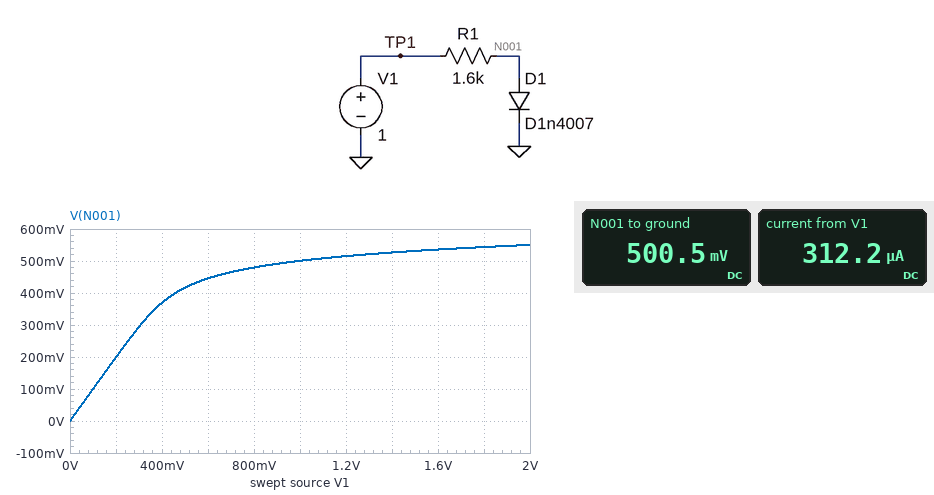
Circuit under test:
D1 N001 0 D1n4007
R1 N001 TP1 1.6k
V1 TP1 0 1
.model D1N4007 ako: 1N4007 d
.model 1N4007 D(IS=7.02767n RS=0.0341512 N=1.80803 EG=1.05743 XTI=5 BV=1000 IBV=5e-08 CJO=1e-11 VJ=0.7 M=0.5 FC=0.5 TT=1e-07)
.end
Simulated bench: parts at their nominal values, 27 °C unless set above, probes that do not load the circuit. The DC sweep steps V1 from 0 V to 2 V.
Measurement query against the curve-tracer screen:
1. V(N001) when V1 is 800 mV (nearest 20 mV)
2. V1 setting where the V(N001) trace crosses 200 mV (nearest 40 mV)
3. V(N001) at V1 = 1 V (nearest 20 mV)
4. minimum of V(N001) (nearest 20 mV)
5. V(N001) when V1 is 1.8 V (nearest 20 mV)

480 mV
200 mV
500 mV
0 V
540 mV
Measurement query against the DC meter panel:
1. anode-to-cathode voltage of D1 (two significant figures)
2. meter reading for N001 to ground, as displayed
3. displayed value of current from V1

500 mV
500.5 mV
312.2 µA
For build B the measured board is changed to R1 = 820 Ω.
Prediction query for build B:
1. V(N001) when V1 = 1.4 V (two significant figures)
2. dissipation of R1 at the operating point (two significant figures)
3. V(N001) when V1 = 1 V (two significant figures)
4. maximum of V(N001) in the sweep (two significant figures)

560 mV
270 µW
530 mV
580 mV
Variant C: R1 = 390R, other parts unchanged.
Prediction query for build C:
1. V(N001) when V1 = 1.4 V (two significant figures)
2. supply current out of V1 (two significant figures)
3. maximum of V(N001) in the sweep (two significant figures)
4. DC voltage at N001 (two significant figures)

590 mV
1.1 mA
610 mV
560 mV
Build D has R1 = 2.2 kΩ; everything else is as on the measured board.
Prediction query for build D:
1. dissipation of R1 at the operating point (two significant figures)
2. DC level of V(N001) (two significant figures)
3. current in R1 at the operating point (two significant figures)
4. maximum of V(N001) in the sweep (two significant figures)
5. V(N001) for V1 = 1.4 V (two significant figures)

120 µW
490 mV
230 µA
540 mV
510 mV
